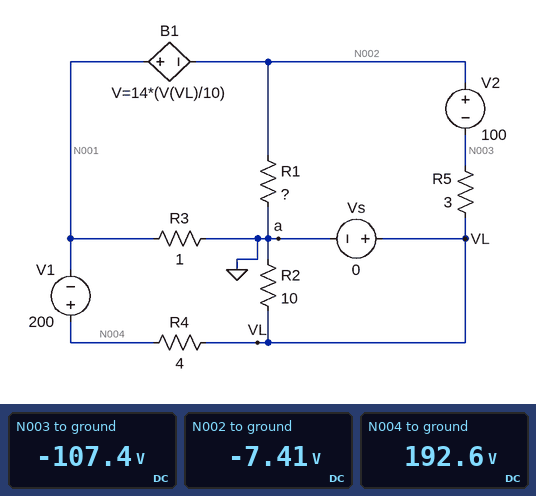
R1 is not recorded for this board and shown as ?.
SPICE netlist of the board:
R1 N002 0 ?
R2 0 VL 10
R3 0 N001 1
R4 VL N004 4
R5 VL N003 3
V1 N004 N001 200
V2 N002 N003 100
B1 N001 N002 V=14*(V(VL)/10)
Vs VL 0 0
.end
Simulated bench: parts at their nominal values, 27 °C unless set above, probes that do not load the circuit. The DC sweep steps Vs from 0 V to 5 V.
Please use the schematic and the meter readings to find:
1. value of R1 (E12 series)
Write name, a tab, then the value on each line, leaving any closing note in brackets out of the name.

value of R1	1.5 Ω
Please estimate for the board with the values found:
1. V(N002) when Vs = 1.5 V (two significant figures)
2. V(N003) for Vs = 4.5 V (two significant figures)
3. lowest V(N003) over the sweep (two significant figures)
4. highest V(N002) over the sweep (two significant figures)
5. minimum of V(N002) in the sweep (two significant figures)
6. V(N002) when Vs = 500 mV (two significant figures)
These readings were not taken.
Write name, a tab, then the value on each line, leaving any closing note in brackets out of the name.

V(N002) when Vs = 1.5 V	-8.2 V
V(N003) for Vs = 4.5 V	-110 V
lowest V(N003) over the sweep	-110 V
highest V(N002) over the sweep	-7.4 V
minimum of V(N002) in the sweep	-10 V
V(N002) when Vs = 500 mV	-7.7 V
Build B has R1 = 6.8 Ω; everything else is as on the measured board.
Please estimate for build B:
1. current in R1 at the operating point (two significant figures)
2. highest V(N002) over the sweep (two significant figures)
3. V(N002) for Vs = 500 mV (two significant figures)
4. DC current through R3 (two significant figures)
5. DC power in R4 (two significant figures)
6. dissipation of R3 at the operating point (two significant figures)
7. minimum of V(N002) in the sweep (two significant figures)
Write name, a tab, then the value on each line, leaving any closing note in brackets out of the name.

current in R1 at the operating point	1.4 A
highest V(N002) over the sweep	-9.6 V
V(N002) for Vs = 500 mV	-10 V
DC current through R3	9.6 A
DC power in R4	9.1 kW
dissipation of R3 at the operating point	93 W
minimum of V(N002) in the sweep	-13 V
